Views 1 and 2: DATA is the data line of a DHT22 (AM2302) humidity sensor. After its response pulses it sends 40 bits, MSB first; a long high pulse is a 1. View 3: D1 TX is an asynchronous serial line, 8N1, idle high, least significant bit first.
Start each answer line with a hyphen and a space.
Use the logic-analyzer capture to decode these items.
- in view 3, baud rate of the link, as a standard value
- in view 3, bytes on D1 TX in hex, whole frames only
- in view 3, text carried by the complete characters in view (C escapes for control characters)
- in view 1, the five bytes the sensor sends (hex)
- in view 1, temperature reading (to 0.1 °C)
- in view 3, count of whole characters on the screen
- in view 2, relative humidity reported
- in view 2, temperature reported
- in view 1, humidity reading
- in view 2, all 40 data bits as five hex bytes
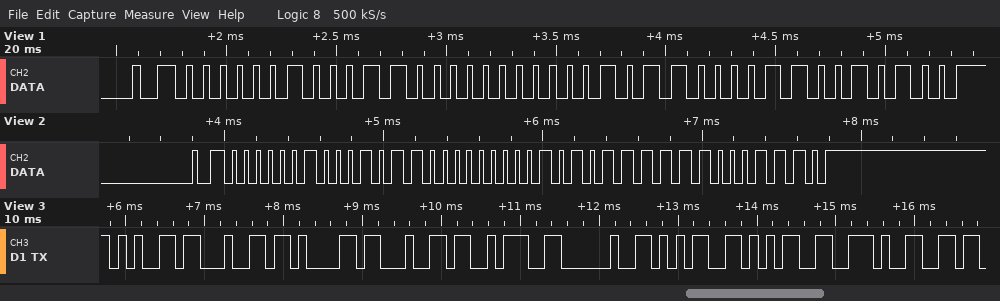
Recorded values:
- 9600 baud
- 65 64 61 64 3A 20 35 35 2E
- "edad: 55."
- 02 30 01 61 94
- 35.3 °C
- 9
- 55.6 %
- 35.1 °C
- 56.0 %
- 02 2C 01 5F 8E
